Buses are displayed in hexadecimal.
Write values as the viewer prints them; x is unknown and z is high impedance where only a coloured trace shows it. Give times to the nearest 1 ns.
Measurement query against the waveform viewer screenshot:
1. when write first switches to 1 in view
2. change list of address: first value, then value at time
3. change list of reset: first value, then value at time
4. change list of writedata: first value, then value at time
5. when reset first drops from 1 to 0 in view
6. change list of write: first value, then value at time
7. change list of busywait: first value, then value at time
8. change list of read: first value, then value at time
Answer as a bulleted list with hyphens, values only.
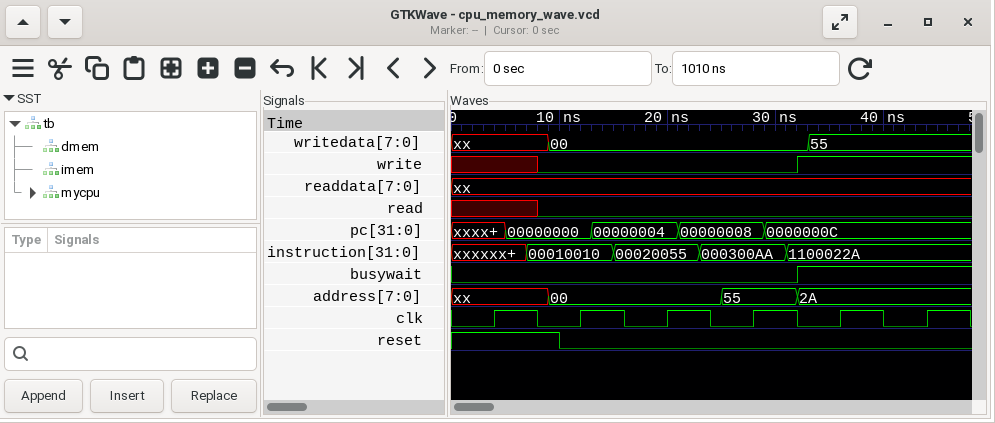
- 32 ns
- xx, 00 at 9 ns, 55 at 25 ns, 2A at 32 ns
- 1, 0 at 10 ns
- xx, 00 at 9 ns, 55 at 33 ns
- 10 ns
- x, 0 at 8 ns, 1 at 32 ns
- 0, 1 at 32 ns
- x, 0 at 8 ns
